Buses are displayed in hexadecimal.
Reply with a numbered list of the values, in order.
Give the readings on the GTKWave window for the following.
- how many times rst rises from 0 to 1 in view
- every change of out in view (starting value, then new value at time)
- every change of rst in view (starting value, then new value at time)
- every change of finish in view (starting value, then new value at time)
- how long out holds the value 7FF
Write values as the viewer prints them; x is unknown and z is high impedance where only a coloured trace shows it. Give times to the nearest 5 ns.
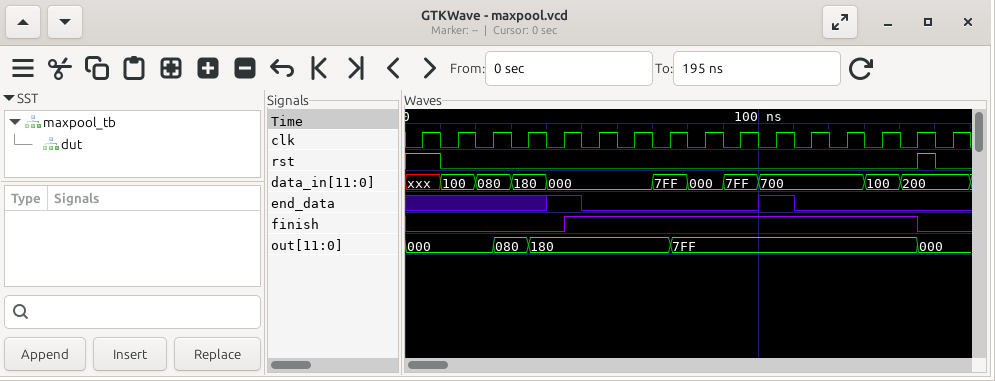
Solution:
1. 1
2. 000, 080 at 25 ns, 180 at 35 ns, 7FF at 75 ns, 000 at 145 ns
3. 1, 0 at 10 ns, 1 at 145 ns, 0 at 150 ns
4. 0, 1 at 45 ns, 0 at 145 ns
5. 70 ns
